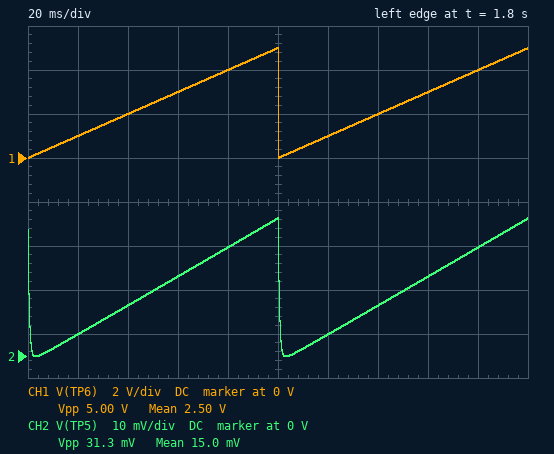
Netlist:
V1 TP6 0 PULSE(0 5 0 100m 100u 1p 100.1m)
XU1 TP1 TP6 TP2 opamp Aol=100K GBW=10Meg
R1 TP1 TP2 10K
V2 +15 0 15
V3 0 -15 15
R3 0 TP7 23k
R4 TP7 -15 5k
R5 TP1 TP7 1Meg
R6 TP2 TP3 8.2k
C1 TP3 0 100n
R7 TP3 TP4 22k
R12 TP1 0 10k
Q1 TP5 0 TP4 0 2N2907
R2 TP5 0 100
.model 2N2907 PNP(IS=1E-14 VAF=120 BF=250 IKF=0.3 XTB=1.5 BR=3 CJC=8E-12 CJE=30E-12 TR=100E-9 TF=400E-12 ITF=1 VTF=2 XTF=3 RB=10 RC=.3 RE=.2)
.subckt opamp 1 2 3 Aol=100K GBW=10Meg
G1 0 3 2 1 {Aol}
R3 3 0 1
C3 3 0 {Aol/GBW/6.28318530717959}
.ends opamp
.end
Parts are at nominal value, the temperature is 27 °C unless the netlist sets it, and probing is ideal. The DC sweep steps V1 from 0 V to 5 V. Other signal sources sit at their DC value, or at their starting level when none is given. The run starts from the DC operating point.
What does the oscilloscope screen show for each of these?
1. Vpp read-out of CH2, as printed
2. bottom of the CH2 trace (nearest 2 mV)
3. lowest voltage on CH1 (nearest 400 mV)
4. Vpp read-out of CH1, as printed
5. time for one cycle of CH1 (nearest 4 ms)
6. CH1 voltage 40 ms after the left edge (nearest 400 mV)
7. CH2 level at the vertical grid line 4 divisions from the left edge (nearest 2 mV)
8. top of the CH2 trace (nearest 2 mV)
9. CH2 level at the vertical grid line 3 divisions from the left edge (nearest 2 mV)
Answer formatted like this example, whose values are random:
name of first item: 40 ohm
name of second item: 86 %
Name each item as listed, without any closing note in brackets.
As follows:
Vpp read-out of CH2, as printed: 31.3 mV
bottom of the CH2 trace: 0 V
lowest voltage on CH1: 0 V
Vpp read-out of CH1, as printed: 5.00 V
time for one cycle of CH1: 100 ms
CH1 voltage 40 ms after the left edge: 2.0 V
CH2 level at the vertical grid line 4 divisions from the left edge: 24 mV
top of the CH2 trace: 32 mV
CH2 level at the vertical grid line 3 divisions from the left edge: 18 mV
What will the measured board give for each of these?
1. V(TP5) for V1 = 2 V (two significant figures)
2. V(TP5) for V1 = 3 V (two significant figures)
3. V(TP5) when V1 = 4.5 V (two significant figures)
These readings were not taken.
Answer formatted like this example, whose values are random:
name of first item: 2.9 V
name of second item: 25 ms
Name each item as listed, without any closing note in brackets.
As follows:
V(TP5) for V1 = 2 V: 12 mV
V(TP5) for V1 = 3 V: 18 mV
V(TP5) when V1 = 4.5 V: 28 mV
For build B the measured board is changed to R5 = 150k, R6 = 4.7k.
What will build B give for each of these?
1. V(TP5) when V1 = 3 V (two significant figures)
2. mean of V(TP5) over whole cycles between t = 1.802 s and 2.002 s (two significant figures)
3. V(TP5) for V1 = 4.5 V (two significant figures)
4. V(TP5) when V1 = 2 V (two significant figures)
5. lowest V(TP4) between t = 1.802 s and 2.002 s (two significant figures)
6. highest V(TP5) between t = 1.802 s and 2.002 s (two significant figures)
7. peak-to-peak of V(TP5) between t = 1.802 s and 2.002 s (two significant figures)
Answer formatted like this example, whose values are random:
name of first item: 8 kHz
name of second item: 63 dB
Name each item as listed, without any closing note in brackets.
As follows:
V(TP5) when V1 = 3 V: 24 mV
mean of V(TP5) over whole cycles between t = 1.802 s and 2.002 s: 20 mV
V(TP5) for V1 = 4.5 V: 35 mV
V(TP5) when V1 = 2 V: 16 mV
lowest V(TP4) between t = 1.802 s and 2.002 s: 550 mV
highest V(TP5) between t = 1.802 s and 2.002 s: 39 mV
peak-to-peak of V(TP5) between t = 1.802 s and 2.002 s: 37 mV
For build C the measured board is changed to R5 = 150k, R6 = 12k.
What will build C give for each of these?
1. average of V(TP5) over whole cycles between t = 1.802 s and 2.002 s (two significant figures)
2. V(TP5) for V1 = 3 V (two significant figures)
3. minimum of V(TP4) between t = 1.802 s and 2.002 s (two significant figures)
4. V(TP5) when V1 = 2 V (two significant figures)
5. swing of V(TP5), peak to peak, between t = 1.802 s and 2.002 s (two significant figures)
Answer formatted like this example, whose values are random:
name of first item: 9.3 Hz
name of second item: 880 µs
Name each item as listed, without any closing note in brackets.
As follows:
average of V(TP5) over whole cycles between t = 1.802 s and 2.002 s: 16 mV
V(TP5) for V1 = 3 V: 19 mV
minimum of V(TP4) between t = 1.802 s and 2.002 s: 550 mV
V(TP5) when V1 = 2 V: 13 mV
swing of V(TP5), peak to peak, between t = 1.802 s and 2.002 s: 29 mV
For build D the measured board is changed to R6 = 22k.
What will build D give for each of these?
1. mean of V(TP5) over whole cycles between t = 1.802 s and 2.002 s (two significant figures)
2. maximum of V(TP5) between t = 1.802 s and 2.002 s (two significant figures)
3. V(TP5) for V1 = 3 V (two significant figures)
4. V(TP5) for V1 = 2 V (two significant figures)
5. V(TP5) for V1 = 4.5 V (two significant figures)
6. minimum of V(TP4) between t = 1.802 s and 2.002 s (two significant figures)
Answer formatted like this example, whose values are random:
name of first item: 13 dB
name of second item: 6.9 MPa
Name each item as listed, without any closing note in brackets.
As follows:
mean of V(TP5) over whole cycles between t = 1.802 s and 2.002 s: 10 mV
maximum of V(TP5) between t = 1.802 s and 2.002 s: 21 mV
V(TP5) for V1 = 3 V: 13 mV
V(TP5) for V1 = 2 V: 8.0 mV
V(TP5) for V1 = 4.5 V: 19 mV
minimum of V(TP4) between t = 1.802 s and 2.002 s: 500 mV
